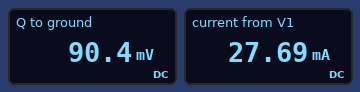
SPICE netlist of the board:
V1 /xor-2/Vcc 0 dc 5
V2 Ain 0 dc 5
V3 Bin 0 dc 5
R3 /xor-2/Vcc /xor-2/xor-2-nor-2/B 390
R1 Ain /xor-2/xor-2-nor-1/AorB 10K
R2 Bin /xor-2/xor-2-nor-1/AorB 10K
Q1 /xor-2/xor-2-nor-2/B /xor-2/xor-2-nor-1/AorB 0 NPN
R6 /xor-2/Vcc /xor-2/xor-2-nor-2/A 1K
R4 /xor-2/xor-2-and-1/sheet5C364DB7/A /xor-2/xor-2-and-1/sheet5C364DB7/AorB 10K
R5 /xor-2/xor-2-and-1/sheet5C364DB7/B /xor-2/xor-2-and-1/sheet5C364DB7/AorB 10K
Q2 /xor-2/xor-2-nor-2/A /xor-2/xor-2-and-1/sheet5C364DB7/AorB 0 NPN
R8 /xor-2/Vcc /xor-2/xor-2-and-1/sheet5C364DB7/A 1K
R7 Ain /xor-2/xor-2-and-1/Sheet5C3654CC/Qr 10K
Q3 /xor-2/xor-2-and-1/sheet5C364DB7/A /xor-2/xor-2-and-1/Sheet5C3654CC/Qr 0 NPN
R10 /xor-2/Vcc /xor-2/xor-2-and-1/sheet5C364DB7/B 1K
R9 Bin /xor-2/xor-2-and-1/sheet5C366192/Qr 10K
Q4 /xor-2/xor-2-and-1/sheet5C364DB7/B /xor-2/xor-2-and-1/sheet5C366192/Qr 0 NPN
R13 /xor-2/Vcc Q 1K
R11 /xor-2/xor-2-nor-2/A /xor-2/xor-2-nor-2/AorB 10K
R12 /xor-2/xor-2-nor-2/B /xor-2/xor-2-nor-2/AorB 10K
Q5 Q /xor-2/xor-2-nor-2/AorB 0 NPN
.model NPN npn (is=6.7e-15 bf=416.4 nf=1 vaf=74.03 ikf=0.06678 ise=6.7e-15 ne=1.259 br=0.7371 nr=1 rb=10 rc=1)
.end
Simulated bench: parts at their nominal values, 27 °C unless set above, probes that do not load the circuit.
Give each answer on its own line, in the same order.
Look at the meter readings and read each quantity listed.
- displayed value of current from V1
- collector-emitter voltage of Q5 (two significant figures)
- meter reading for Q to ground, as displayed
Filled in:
27.69 mA
90 mV
90.4 mV
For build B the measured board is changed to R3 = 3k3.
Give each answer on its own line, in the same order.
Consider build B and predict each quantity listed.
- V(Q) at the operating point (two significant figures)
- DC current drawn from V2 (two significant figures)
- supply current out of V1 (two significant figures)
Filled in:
91 mV
860 µA
17 mA
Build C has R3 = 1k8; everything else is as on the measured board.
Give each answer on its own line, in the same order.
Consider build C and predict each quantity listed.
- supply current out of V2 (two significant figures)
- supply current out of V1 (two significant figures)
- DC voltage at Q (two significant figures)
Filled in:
860 µA
18 mA
91 mV
